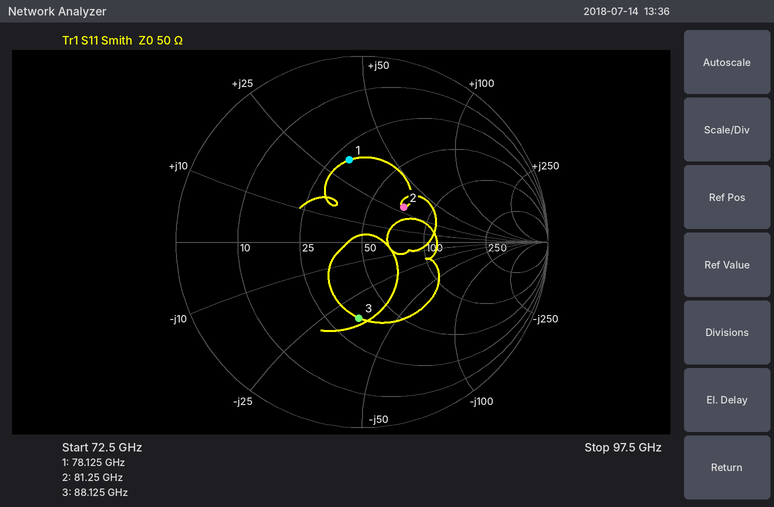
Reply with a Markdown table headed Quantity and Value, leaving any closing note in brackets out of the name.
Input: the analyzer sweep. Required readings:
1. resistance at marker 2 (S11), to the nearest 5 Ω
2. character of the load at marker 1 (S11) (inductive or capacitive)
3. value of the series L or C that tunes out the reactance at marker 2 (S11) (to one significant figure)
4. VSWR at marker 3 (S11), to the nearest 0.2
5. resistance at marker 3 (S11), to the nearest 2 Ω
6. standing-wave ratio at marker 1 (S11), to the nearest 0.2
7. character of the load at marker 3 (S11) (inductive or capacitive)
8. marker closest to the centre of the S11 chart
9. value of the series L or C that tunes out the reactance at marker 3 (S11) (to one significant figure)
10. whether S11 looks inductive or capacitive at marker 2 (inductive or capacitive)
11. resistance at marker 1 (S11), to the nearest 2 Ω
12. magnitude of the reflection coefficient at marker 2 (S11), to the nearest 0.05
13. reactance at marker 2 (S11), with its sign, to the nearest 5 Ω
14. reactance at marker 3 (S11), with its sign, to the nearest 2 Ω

| Quantity | Value |
|---|---|
| resistance at marker 2 (S11), to the nearest 5 Ω | 70 Ω |
| character of the load at marker 1 (S11) | inductive |
| value of the series L or C that tunes out the reactance at marker 2 (S11) | 70 fF |
| VSWR at marker 3 (S11), to the nearest 0.2 | 2.4 |
| resistance at marker 3 (S11), to the nearest 2 Ω | 34 Ω |
| standing-wave ratio at marker 1 (S11), to the nearest 0.2 | 2.6 |
| character of the load at marker 3 (S11) | capacitive |
| marker closest to the centre of the S11 chart | marker 2 |
| value of the series L or C that tunes out the reactance at marker 3 (S11) | 60 pH |
| whether S11 looks inductive or capacitive at marker 2 | inductive |
| resistance at marker 1 (S11), to the nearest 2 Ω | 30 Ω |
| magnitude of the reflection coefficient at marker 2 (S11), to the nearest 0.05 | 0.30 |
| reactance at marker 2 (S11), with its sign, to the nearest 5 Ω | +30 Ω |
| reactance at marker 3 (S11), with its sign, to the nearest 2 Ω | -34 Ω |
